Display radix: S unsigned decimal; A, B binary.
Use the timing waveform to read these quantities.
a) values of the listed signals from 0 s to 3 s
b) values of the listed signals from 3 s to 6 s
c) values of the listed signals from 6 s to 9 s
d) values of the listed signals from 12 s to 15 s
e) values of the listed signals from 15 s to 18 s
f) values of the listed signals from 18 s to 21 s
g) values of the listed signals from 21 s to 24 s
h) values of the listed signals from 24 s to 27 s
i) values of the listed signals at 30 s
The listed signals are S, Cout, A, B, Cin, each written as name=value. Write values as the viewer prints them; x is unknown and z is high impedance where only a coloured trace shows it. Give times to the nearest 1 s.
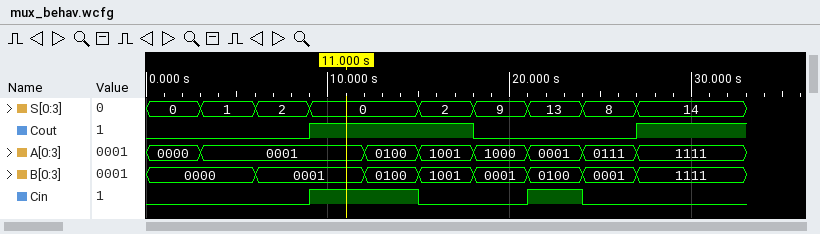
S=0, Cout=0, A=0000, B=0000, Cin=0
S=1, Cout=0, A=0001, B=0000, Cin=0
S=2, Cout=0, A=0001, B=0001, Cin=0
S=0, Cout=1, A=0100, B=0100, Cin=1
S=2, Cout=1, A=1001, B=1001, Cin=0
S=9, Cout=0, A=1000, B=0001, Cin=0
S=13, Cout=0, A=0001, B=0100, Cin=1
S=8, Cout=0, A=0111, B=0001, Cin=0
S=14, Cout=1, A=1111, B=1111, Cin=0
